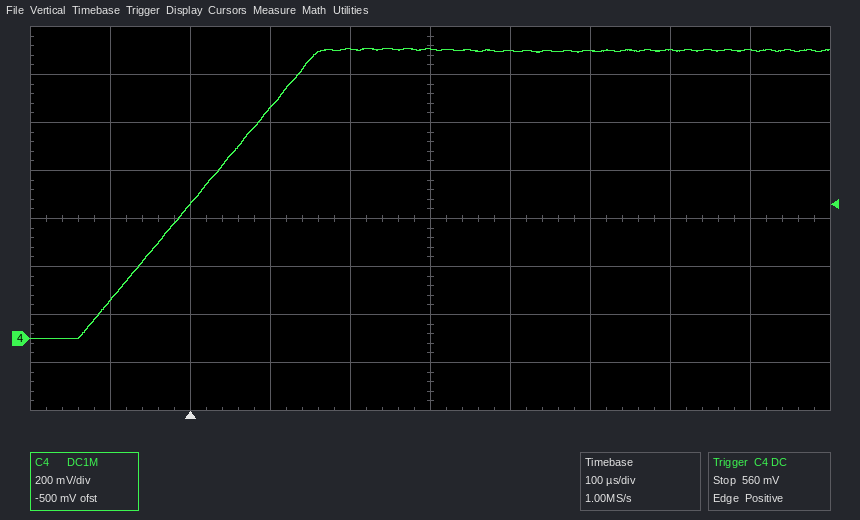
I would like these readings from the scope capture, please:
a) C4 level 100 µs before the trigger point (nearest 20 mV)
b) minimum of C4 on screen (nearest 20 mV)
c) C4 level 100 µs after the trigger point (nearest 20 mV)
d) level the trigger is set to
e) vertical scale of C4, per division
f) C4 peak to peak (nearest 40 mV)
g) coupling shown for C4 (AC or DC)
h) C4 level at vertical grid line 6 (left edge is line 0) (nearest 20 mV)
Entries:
160 mV
0 mV
960 mV
560 mV
200 mV
1.20 V
DC
1.20 V
